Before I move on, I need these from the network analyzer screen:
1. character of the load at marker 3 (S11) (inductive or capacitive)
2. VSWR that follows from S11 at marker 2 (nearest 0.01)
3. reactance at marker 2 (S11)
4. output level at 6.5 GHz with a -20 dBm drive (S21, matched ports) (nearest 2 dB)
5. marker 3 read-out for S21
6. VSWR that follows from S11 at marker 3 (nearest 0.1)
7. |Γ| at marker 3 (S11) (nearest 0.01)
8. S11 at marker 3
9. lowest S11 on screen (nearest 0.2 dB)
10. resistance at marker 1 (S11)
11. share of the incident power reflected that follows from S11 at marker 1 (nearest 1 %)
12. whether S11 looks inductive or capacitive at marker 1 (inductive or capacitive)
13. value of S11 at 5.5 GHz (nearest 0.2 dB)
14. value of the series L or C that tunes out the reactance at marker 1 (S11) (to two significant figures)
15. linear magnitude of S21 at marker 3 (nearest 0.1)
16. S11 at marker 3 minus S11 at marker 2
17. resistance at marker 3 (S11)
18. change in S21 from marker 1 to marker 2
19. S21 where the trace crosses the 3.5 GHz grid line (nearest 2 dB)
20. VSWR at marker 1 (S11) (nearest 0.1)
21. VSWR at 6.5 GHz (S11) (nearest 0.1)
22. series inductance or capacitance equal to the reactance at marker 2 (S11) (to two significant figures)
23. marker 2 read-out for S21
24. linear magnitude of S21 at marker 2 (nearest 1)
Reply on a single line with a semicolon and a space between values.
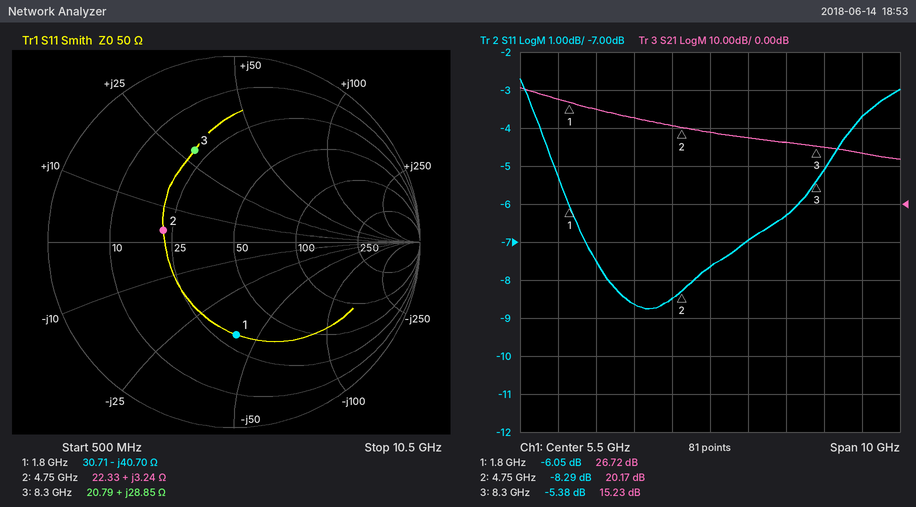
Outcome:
inductive; 2.25; +3.24 Ω; -2 dBm; 15.23 dB; 3.3; 0.54; -5.38 dB; -8.8 dB; 30.71 Ω; 25 %; capacitive; -7.6 dB; 3.6 nH; 5.8; 2.91 dB; 20.79 Ω; -6.55 dB; 22 dB; 3.0; 2.6; 110 pH; 20.17 dB; 10
